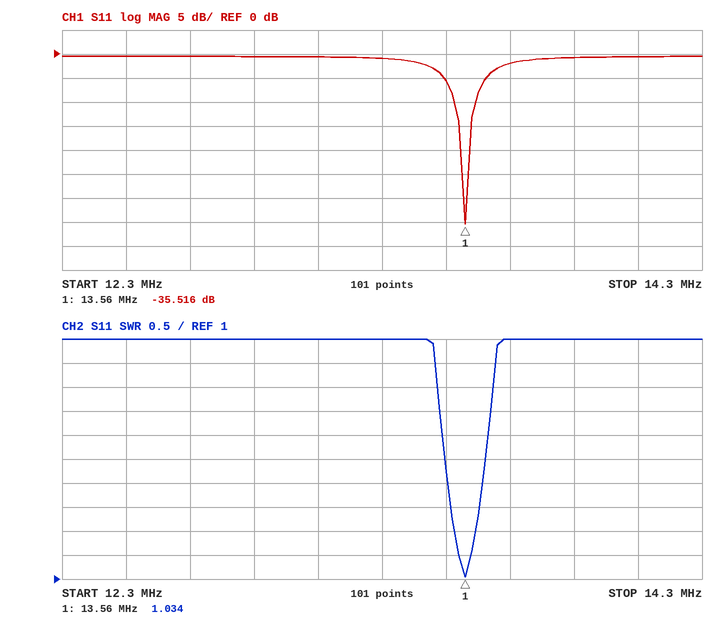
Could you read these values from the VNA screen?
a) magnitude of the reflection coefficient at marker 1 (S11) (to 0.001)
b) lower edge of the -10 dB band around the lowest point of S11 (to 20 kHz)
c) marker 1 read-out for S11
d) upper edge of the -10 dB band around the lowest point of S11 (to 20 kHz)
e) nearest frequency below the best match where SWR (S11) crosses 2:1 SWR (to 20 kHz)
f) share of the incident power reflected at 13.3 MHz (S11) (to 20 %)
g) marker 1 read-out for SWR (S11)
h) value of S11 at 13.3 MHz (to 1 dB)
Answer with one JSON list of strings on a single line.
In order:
["0.017", "13.52 MHz", "-35.516 dB", "13.60 MHz", "13.52 MHz", "80 %", "1.034", "-1 dB"]
